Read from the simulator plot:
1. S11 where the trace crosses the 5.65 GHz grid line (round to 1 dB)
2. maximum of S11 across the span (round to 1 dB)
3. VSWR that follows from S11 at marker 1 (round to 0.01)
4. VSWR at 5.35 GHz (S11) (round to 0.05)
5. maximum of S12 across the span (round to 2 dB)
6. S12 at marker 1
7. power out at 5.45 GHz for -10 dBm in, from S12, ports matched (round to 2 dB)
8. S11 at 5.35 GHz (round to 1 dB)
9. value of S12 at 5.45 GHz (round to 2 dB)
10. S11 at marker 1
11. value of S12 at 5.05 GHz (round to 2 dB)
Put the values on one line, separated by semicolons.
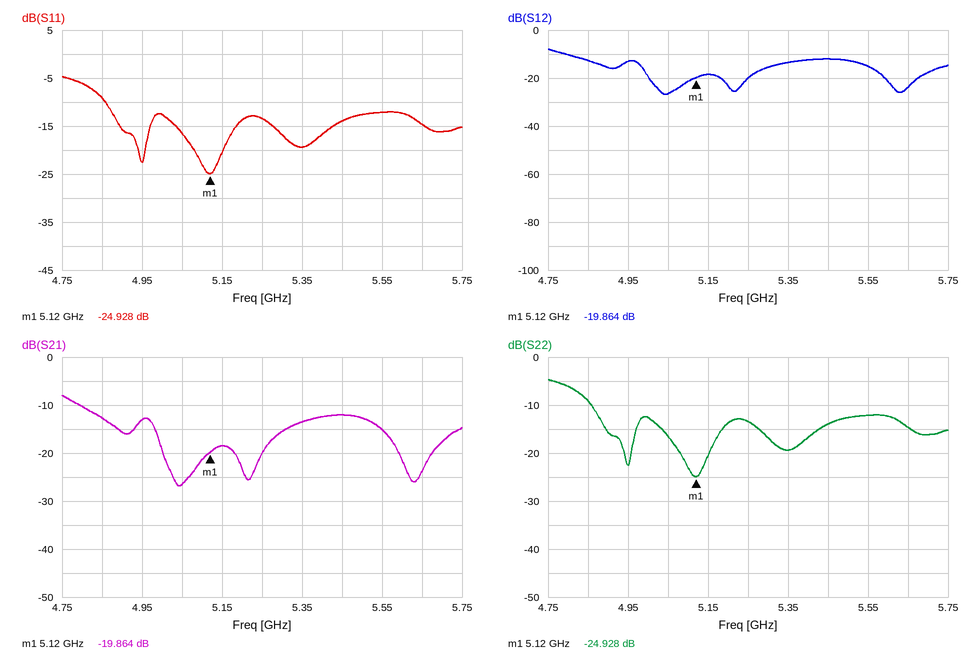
-15 dB; -5 dB; 1.12; 1.25; -8 dB; -19.864 dB; -22 dBm; -19 dB; -12 dB; -24.928 dB; -26 dB
